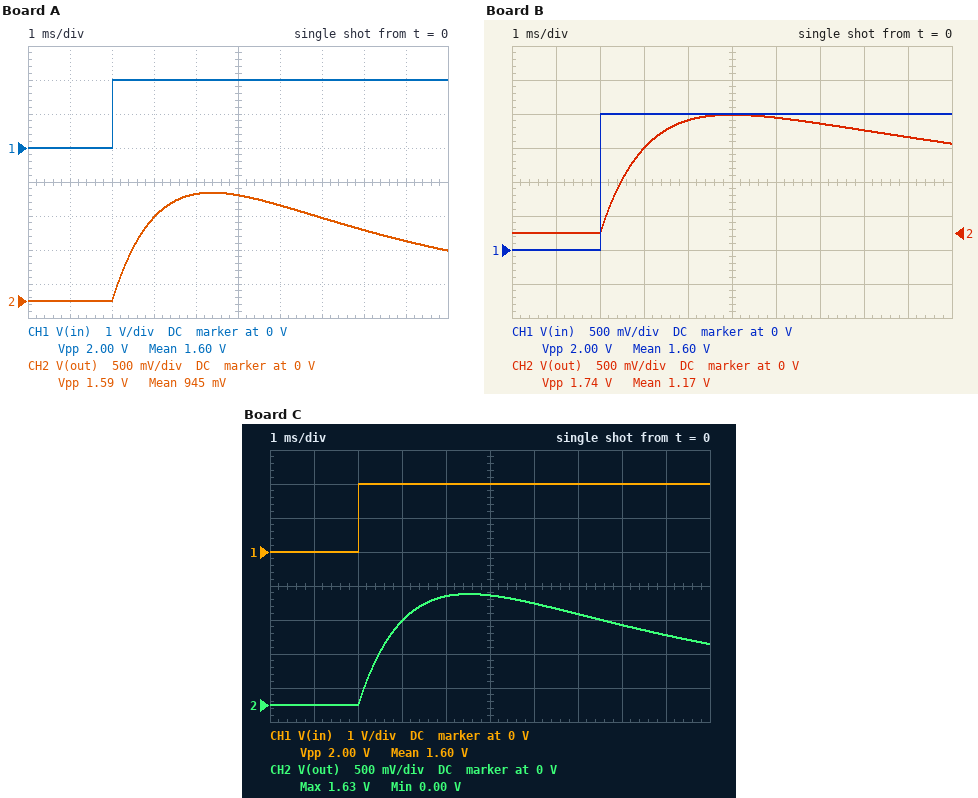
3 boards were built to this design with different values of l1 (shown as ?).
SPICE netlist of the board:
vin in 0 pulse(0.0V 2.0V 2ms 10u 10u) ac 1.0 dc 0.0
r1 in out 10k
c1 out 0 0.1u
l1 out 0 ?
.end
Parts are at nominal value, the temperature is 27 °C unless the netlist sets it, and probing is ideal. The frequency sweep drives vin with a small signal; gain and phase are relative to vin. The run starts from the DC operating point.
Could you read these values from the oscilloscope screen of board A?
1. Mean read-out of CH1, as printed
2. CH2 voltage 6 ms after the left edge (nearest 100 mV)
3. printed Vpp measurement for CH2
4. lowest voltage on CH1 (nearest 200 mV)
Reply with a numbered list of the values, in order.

1. 1.60 V
2. 1.4 V
3. 1.59 V
4. 0 V
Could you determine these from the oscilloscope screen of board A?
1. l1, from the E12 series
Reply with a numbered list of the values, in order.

1. 68 H
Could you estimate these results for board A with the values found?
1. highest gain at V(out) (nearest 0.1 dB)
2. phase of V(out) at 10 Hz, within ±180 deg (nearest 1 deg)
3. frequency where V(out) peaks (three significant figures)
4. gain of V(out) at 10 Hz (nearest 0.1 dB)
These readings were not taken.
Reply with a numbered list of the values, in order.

1. 0 dB
2. 66 deg
3. 61.0 Hz
4. -7.9 dB
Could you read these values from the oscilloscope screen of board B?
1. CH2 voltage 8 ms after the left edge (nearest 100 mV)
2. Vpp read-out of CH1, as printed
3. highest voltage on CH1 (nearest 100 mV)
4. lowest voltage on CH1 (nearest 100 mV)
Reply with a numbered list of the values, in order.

1. 1.5 V
2. 2.00 V
3. 2.0 V
4. 0 V
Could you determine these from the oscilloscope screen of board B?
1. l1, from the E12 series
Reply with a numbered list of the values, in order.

1. 150 H
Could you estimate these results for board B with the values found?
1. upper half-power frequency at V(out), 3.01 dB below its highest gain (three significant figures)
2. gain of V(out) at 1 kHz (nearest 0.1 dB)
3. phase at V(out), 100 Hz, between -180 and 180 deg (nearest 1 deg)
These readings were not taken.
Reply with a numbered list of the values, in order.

1. 169 Hz
2. -16.1 dB
3. -28 deg
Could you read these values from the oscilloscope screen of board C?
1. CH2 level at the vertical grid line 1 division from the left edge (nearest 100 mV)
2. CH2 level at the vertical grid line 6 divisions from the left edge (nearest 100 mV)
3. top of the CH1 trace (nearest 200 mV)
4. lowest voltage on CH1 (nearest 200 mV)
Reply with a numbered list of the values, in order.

1. 0 V
2. 1.5 V
3. 2.0 V
4. 0 V
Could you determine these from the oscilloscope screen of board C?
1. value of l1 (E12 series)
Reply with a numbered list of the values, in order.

1. 82 H
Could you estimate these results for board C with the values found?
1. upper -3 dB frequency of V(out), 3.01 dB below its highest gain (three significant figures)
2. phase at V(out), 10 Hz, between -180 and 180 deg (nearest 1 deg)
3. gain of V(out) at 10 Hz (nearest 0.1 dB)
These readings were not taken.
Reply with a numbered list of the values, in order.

1. 177 Hz
2. 62 deg
3. -6.6 dB
